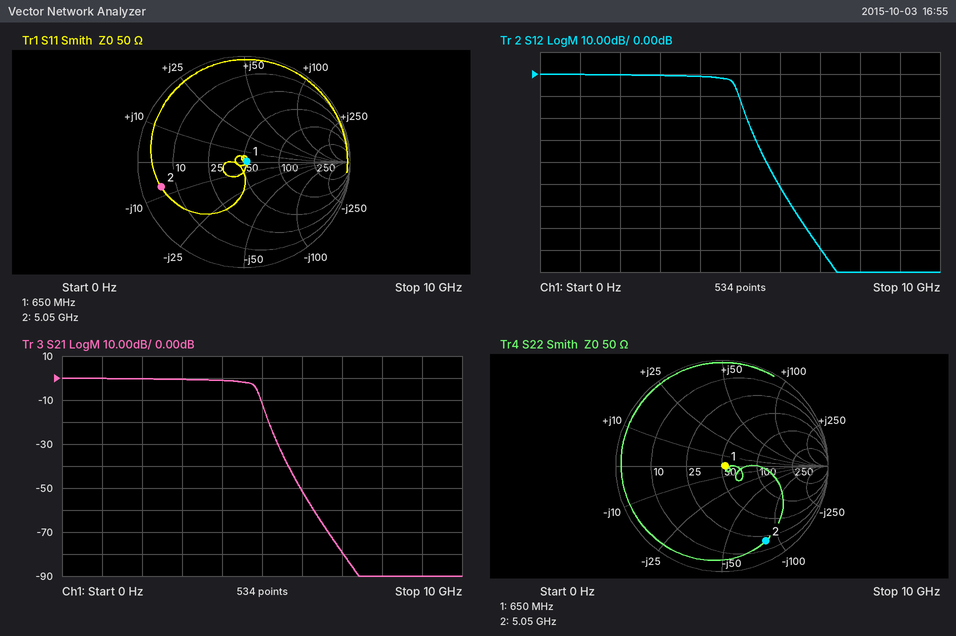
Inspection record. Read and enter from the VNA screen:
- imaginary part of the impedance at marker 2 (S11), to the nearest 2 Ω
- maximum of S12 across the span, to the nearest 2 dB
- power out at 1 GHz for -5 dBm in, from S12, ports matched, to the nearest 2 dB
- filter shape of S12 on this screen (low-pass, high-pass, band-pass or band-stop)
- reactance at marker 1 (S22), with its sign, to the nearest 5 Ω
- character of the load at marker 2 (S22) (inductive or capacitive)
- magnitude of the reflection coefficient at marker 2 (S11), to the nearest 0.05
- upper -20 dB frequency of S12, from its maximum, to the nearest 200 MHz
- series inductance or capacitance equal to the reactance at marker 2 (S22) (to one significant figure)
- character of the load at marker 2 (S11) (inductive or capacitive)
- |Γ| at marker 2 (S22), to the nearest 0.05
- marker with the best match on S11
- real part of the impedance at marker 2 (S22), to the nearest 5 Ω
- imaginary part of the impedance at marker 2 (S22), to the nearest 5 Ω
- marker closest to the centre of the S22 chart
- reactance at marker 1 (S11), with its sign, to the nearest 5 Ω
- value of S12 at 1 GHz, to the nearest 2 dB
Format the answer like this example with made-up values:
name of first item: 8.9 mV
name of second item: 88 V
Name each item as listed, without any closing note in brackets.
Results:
imaginary part of the impedance at marker 2 (S11), to the nearest 2 Ω: -8 Ω
maximum of S12 across the span, to the nearest 2 dB: 0 dB
power out at 1 GHz for -5 dBm in, from S12, ports matched, to the nearest 2 dB: -6 dBm
filter shape of S12 on this screen: low-pass
reactance at marker 1 (S22), with its sign, to the nearest 5 Ω: 0 Ω
character of the load at marker 2 (S22): capacitive
magnitude of the reflection coefficient at marker 2 (S11), to the nearest 0.05: 0.80
upper -20 dB frequency of S12, from its maximum, to the nearest 200 MHz: 5.2 GHz
series inductance or capacitance equal to the reactance at marker 2 (S22): 400 fF
character of the load at marker 2 (S11): capacitive
|Γ| at marker 2 (S22), to the nearest 0.05: 0.80
marker with the best match on S11: marker 1
real part of the impedance at marker 2 (S22), to the nearest 5 Ω: 20 Ω
imaginary part of the impedance at marker 2 (S22), to the nearest 5 Ω: -85 Ω
marker closest to the centre of the S22 chart: marker 1
reactance at marker 1 (S11), with its sign, to the nearest 5 Ω: 0 Ω
value of S12 at 1 GHz, to the nearest 2 dB: 0 dB
